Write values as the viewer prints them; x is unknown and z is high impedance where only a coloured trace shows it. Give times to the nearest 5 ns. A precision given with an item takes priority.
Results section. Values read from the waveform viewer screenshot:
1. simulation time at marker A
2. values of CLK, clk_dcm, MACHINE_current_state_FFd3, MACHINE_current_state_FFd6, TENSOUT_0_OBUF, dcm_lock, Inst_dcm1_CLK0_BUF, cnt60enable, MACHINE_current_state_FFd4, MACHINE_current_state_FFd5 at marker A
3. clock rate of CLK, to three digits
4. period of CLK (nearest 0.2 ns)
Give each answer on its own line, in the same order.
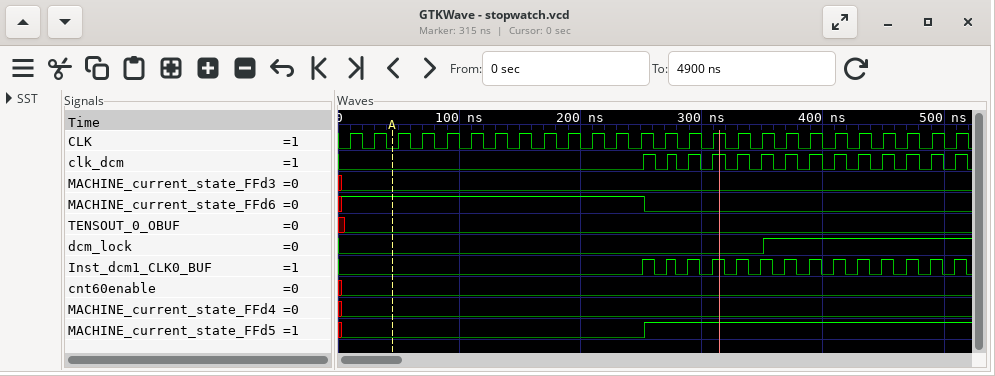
45 ns
CLK=0, clk_dcm=0, MACHINE_current_state_FFd3=0, MACHINE_current_state_FFd6=1, TENSOUT_0_OBUF=0, dcm_lock=0, Inst_dcm1_CLK0_BUF=0, cnt60enable=0, MACHINE_current_state_FFd4=0, MACHINE_current_state_FFd5=0
50.0 MHz
20 ns
